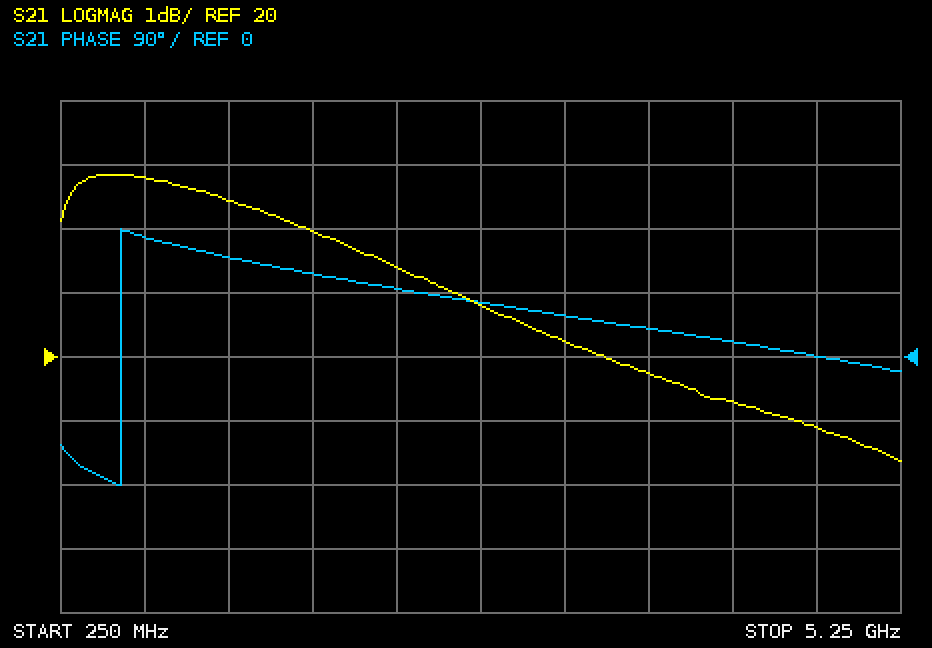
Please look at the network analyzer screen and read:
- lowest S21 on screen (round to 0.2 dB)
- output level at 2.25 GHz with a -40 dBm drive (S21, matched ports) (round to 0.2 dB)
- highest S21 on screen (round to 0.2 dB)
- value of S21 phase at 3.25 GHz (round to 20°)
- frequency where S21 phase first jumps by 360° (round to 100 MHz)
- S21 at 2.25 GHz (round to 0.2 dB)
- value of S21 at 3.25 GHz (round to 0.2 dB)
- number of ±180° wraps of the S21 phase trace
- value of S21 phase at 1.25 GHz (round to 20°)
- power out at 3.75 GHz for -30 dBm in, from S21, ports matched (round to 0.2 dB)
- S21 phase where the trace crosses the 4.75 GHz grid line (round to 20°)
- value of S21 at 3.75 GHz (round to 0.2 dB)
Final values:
18.4 dB
-18.6 dBm
22.8 dB
60°
600 MHz
21.4 dB
20.2 dB
1
140°
-10.2 dBm
0°
19.8 dB
